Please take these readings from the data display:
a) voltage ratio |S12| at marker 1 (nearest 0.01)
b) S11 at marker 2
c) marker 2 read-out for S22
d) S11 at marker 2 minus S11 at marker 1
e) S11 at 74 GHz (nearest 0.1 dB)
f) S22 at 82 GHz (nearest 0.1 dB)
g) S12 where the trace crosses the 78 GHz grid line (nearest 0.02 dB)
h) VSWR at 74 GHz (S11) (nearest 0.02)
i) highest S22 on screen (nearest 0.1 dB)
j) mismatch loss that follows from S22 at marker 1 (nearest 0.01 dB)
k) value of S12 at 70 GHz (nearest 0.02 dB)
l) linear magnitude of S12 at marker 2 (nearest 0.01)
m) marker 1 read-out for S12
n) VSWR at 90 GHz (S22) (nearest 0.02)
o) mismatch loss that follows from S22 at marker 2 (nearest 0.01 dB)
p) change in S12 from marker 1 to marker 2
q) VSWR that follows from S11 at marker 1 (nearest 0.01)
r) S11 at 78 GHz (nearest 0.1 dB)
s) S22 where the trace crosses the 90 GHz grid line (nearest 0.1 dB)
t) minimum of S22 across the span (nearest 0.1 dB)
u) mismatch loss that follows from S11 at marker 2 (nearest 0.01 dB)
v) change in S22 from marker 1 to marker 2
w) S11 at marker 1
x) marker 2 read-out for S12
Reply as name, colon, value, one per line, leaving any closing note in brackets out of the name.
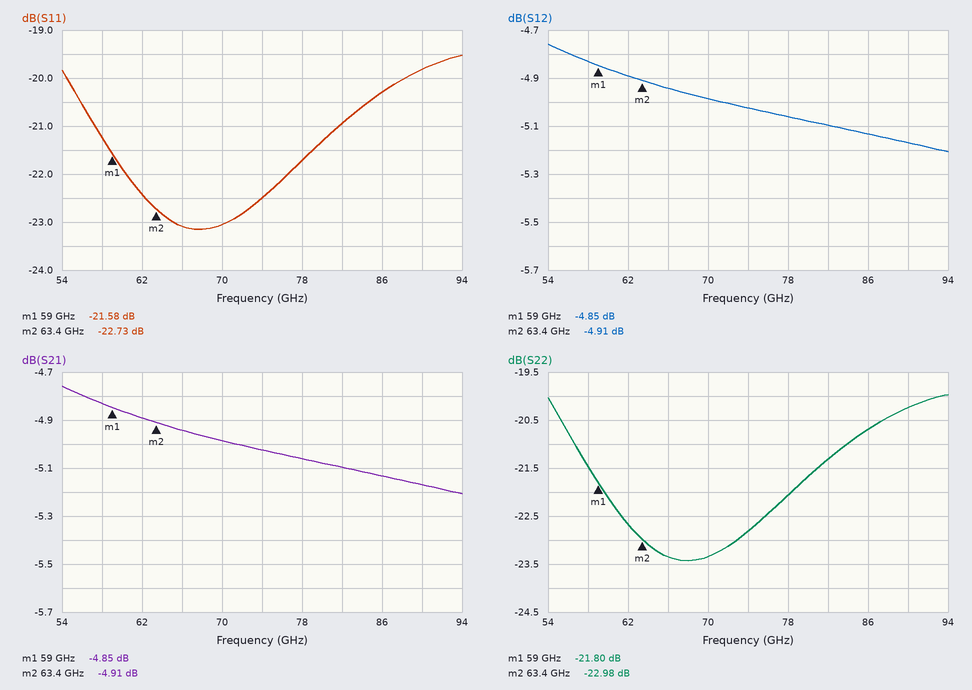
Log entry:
voltage ratio |S12| at marker 1: 0.57
S11 at marker 2: -22.73 dB
marker 2 read-out for S22: -22.98 dB
S11 at marker 2 minus S11 at marker 1: -1.15 dB
S11 at 74 GHz: -22.5 dB
S22 at 82 GHz: -21.3 dB
S12 where the trace crosses the 78 GHz grid line: -5.06 dB
VSWR at 74 GHz (S11): 1.16
highest S22 on screen: -20.0 dB
mismatch loss that follows from S22 at marker 1: 0.03 dB
value of S12 at 70 GHz: -4.98 dB
linear magnitude of S12 at marker 2: 0.57
marker 1 read-out for S12: -4.85 dB
VSWR at 90 GHz (S22): 1.22
mismatch loss that follows from S22 at marker 2: 0.02 dB
change in S12 from marker 1 to marker 2: -0.06 dB
VSWR that follows from S11 at marker 1: 1.18
S11 at 78 GHz: -21.7 dB
S22 where the trace crosses the 90 GHz grid line: -20.2 dB
minimum of S22 across the span: -23.4 dB
mismatch loss that follows from S11 at marker 2: 0.02 dB
change in S22 from marker 1 to marker 2: -1.18 dB
S11 at marker 1: -21.58 dB
marker 2 read-out for S12: -4.91 dB
